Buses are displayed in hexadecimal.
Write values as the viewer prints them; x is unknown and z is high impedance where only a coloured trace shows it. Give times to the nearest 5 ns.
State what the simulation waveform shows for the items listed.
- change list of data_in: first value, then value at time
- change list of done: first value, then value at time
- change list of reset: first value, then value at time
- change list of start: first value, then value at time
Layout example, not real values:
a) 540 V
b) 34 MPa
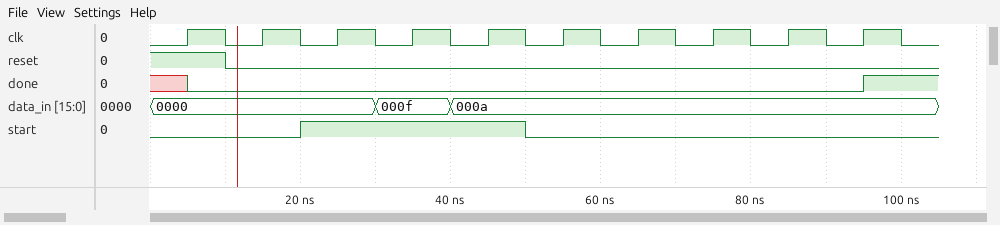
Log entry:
a) 0000, 000f at 30 ns, 000a at 40 ns
b) x, 0 at 5 ns, 1 at 95 ns
c) 1, 0 at 10 ns
d) 0, 1 at 20 ns, 0 at 50 ns
